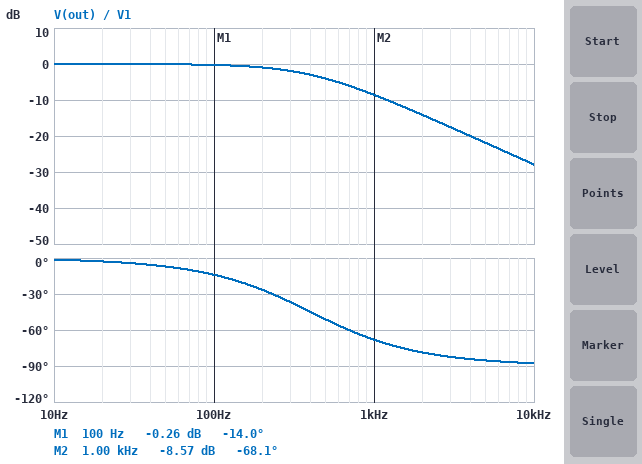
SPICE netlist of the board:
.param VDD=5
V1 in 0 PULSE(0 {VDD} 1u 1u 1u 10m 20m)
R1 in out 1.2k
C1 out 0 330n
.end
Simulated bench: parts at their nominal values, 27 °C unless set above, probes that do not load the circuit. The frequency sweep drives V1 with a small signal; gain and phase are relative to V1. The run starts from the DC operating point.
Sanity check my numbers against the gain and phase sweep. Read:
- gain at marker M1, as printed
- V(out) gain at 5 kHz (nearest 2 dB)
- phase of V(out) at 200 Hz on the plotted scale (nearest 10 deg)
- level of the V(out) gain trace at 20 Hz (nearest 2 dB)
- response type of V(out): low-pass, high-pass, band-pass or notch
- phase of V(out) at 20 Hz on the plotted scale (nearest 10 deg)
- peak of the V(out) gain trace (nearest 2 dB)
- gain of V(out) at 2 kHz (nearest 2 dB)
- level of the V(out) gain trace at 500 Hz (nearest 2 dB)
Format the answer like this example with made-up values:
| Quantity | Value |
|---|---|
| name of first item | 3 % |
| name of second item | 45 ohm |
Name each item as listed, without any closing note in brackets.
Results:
| Quantity | Value |
|---|---|
| gain at marker M1, as printed | -0.26 dB |
| V(out) gain at 5 kHz | -22 dB |
| phase of V(out) at 200 Hz on the plotted scale | -30 deg |
| level of the V(out) gain trace at 20 Hz | 0 dB |
| response type of V(out): low-pass, high-pass, band-pass or notch | low-pass |
| phase of V(out) at 20 Hz on the plotted scale | 0 deg |
| peak of the V(out) gain trace | 0 dB |
| gain of V(out) at 2 kHz | -14 dB |
| level of the V(out) gain trace at 500 Hz | -4 dB |
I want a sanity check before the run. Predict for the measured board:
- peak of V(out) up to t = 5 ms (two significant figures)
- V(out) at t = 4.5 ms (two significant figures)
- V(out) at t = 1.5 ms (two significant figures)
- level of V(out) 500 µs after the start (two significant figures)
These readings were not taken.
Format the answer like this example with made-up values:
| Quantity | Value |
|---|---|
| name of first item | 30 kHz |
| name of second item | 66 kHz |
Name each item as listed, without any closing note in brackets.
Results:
| Quantity | Value |
|---|---|
| peak of V(out) up to t = 5 ms | 5.0 V |
| V(out) at t = 4.5 ms | 5.0 V |
| V(out) at t = 1.5 ms | 4.9 V |
| level of V(out) 500 µs after the start | 3.6 V |
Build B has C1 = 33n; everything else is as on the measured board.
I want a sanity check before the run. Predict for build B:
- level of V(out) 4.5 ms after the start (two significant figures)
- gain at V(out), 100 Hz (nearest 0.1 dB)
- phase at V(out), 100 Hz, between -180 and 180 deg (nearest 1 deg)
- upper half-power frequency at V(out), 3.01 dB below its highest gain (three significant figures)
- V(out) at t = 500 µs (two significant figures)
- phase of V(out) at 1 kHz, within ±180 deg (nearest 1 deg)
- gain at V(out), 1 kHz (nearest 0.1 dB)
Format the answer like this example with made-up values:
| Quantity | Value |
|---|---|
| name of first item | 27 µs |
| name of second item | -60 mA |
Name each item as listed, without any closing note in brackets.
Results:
| Quantity | Value |
|---|---|
| level of V(out) 4.5 ms after the start | 5.0 V |
| gain at V(out), 100 Hz | 0 dB |
| phase at V(out), 100 Hz, between -180 and 180 deg | -1 deg |
| upper half-power frequency at V(out), 3.01 dB below its highest gain | 4.02 kHz |
| V(out) at t = 500 µs | 5.0 V |
| phase of V(out) at 1 kHz, within ±180 deg | -14 deg |
| gain at V(out), 1 kHz | -0.3 dB |
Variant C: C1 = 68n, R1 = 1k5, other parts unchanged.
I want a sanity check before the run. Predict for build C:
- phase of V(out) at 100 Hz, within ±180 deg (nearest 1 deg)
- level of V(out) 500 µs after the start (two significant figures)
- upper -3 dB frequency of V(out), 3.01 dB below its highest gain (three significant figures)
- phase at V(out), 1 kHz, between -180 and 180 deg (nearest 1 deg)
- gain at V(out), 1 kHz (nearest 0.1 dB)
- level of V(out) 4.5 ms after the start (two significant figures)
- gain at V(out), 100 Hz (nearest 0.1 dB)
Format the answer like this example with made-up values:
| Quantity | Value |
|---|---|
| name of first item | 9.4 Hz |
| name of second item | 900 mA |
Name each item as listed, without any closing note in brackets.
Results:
| Quantity | Value |
|---|---|
| phase of V(out) at 100 Hz, within ±180 deg | -4 deg |
| level of V(out) 500 µs after the start | 5.0 V |
| upper -3 dB frequency of V(out), 3.01 dB below its highest gain | 1.56 kHz |
| phase at V(out), 1 kHz, between -180 and 180 deg | -33 deg |
| gain at V(out), 1 kHz | -1.5 dB |
| level of V(out) 4.5 ms after the start | 5.0 V |
| gain at V(out), 100 Hz | 0 dB |
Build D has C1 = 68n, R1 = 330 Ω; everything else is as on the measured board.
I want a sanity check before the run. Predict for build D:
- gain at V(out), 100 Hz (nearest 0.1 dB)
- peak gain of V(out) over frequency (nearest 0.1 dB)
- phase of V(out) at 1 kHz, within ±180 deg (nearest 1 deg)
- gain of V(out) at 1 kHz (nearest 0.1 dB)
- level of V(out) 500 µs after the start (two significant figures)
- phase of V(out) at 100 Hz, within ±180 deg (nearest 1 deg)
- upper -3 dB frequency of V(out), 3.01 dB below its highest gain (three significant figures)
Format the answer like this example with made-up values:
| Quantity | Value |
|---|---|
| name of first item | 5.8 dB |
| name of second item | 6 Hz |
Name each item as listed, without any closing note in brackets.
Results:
| Quantity | Value |
|---|---|
| gain at V(out), 100 Hz | 0 dB |
| peak gain of V(out) over frequency | 0 dB |
| phase of V(out) at 1 kHz, within ±180 deg | -8 deg |
| gain of V(out) at 1 kHz | -0.1 dB |
| level of V(out) 500 µs after the start | 5.0 V |
| phase of V(out) at 100 Hz, within ±180 deg | -1 deg |
| upper -3 dB frequency of V(out), 3.01 dB below its highest gain | 7.09 kHz |
